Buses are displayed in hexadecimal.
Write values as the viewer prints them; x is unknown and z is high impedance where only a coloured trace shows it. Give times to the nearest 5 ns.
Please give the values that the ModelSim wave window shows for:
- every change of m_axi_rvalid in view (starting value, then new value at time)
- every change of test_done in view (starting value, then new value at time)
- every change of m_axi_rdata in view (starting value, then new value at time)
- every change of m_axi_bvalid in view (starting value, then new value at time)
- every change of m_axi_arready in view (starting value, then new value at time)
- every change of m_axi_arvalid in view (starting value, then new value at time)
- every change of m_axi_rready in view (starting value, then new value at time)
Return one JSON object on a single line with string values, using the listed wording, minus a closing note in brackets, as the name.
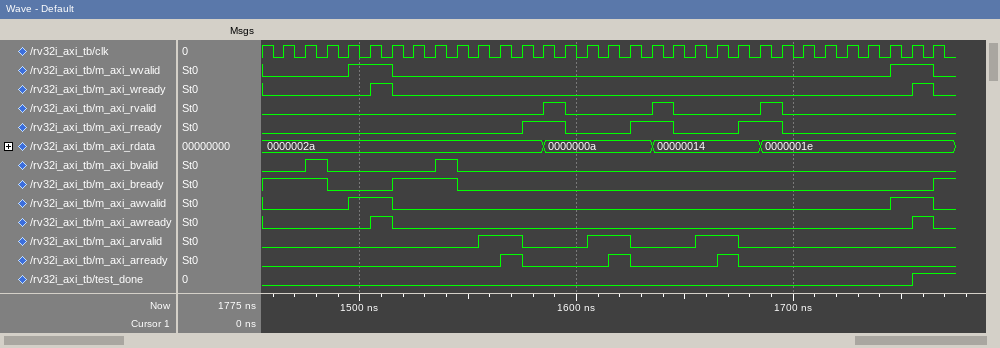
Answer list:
{"every change of m_axi_rvalid in view": "0, 1 at 1585 ns, 0 at 1595 ns, 1 at 1635 ns, 0 at 1645 ns, 1 at 1685 ns, 0 at 1695 ns", "every change of test_done in view": "0, 1 at 1755 ns", "every change of m_axi_rdata in view": "0000002a, 0000000a at 1585 ns, 00000014 at 1635 ns, 0000001e at 1685 ns", "every change of m_axi_bvalid in view": "0, 1 at 1475 ns, 0 at 1485 ns, 1 at 1535 ns, 0 at 1545 ns", "every change of m_axi_arready in view": "0, 1 at 1565 ns, 0 at 1575 ns, 1 at 1615 ns, 0 at 1625 ns, 1 at 1665 ns, 0 at 1675 ns", "every change of m_axi_arvalid in view": "0, 1 at 1555 ns, 0 at 1575 ns, 1 at 1605 ns, 0 at 1625 ns, 1 at 1655 ns, 0 at 1675 ns", "every change of m_axi_rready in view": "0, 1 at 1575 ns, 0 at 1595 ns, 1 at 1625 ns, 0 at 1645 ns, 1 at 1675 ns, 0 at 1695 ns"}
